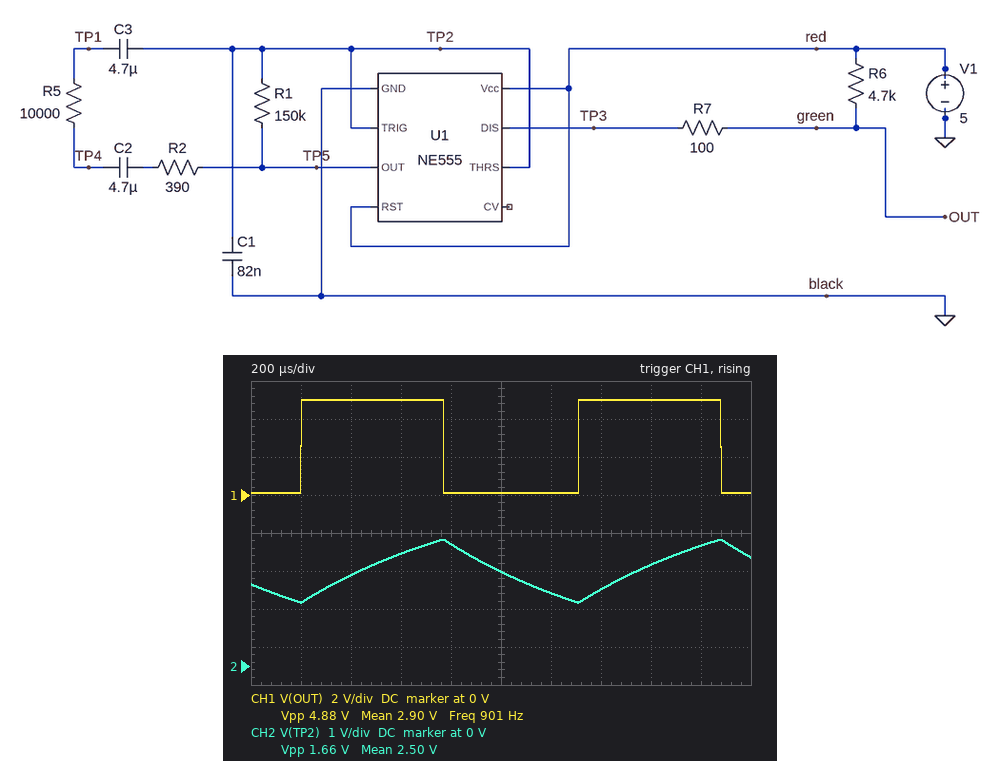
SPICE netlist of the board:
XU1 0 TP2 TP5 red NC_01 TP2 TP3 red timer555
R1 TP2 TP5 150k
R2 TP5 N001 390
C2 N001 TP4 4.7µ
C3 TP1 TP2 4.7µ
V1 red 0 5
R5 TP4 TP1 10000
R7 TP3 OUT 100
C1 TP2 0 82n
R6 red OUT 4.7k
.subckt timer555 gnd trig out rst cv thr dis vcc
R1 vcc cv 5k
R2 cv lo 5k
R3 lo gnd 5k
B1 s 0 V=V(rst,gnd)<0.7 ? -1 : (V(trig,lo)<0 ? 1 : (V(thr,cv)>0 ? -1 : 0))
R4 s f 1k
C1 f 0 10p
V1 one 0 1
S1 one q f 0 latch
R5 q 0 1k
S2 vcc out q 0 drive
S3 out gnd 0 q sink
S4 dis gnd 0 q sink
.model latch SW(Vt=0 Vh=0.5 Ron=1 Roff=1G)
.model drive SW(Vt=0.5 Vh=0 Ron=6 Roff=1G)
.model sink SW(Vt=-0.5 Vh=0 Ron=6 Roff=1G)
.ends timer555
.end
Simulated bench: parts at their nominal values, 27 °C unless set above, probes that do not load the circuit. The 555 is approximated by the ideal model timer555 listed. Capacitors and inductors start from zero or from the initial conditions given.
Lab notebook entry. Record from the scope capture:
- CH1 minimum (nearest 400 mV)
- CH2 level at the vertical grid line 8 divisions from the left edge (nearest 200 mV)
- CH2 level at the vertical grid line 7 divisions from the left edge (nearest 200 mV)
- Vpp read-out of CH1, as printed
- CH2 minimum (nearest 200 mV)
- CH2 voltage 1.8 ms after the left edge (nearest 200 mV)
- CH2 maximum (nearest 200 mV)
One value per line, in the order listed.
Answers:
0 V
2.6 V
2.0 V
4.88 V
1.6 V
3.2 V
3.4 V
